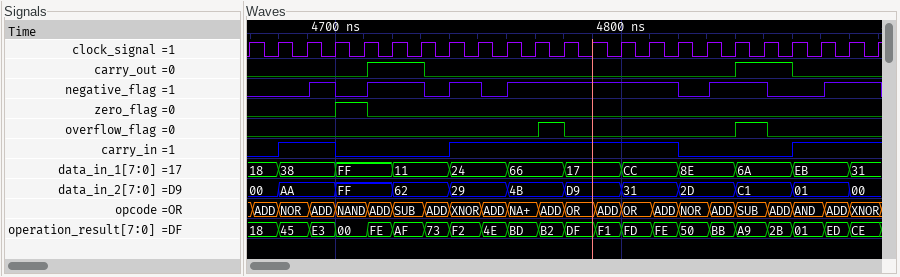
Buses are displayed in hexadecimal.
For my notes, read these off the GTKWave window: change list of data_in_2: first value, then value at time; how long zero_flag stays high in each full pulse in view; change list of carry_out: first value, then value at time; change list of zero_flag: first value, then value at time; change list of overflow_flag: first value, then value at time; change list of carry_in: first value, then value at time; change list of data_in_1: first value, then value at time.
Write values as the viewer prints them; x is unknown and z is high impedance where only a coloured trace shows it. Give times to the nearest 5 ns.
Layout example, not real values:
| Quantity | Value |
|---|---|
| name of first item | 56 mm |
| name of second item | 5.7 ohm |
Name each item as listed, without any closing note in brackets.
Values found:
| Quantity | Value |
|---|---|
| change list of data_in_2: first value, then value at time | 00, AA at 4680 ns, FF at 4700 ns, 62 at 4720 ns, 29 at 4740 ns, 4B at 4760 ns, D9 at 4780 ns, 31 at 4800 ns, 2D at 4820 ns, C1 at 4840 ns, 01 at 4860 ns, 00 at 4880 ns |
| how long zero_flag stays high in each full pulse in view | 10 ns |
| change list of carry_out: first value, then value at time | 0, 1 at 4710 ns, 0 at 4730 ns, 1 at 4840 ns, 0 at 4860 ns |
| change list of zero_flag: first value, then value at time | 0, 1 at 4700 ns, 0 at 4710 ns |
| change list of overflow_flag: first value, then value at time | 0, 1 at 4770 ns, 0 at 4780 ns, 1 at 4840 ns, 0 at 4850 ns |
| change list of carry_in: first value, then value at time | 0, 1 at 4680 ns, 0 at 4700 ns, 1 at 4740 ns, 0 at 4820 ns, 1 at 4860 ns |
| change list of data_in_1: first value, then value at time | 18, 38 at 4680 ns, FF at 4700 ns, 11 at 4720 ns, 24 at 4740 ns, 66 at 4760 ns, 17 at 4780 ns, CC at 4800 ns, 8E at 4820 ns, 6A at 4840 ns, EB at 4860 ns, 31 at 4880 ns |
